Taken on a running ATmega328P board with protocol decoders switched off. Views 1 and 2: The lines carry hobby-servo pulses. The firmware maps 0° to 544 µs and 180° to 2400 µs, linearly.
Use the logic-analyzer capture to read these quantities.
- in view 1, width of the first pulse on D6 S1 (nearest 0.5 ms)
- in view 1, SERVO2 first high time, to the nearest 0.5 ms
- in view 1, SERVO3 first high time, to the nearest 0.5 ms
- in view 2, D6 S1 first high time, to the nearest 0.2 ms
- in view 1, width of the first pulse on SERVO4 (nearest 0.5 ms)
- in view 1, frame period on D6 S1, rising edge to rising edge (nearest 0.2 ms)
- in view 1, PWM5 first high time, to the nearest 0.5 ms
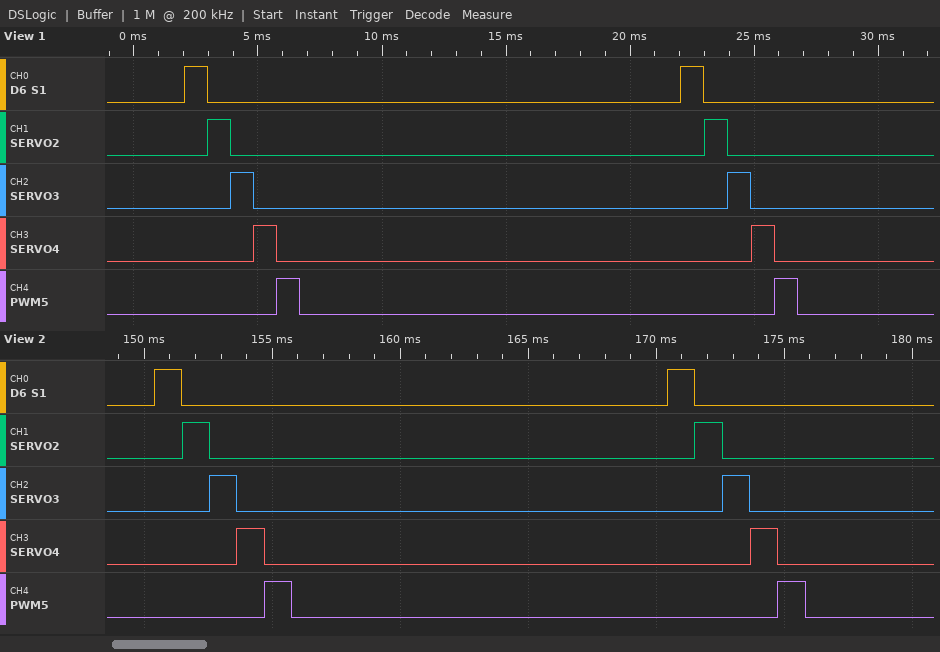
1.0 ms
1.0 ms
1.0 ms
1.0 ms
1.0 ms
20.0 ms
1.0 ms
